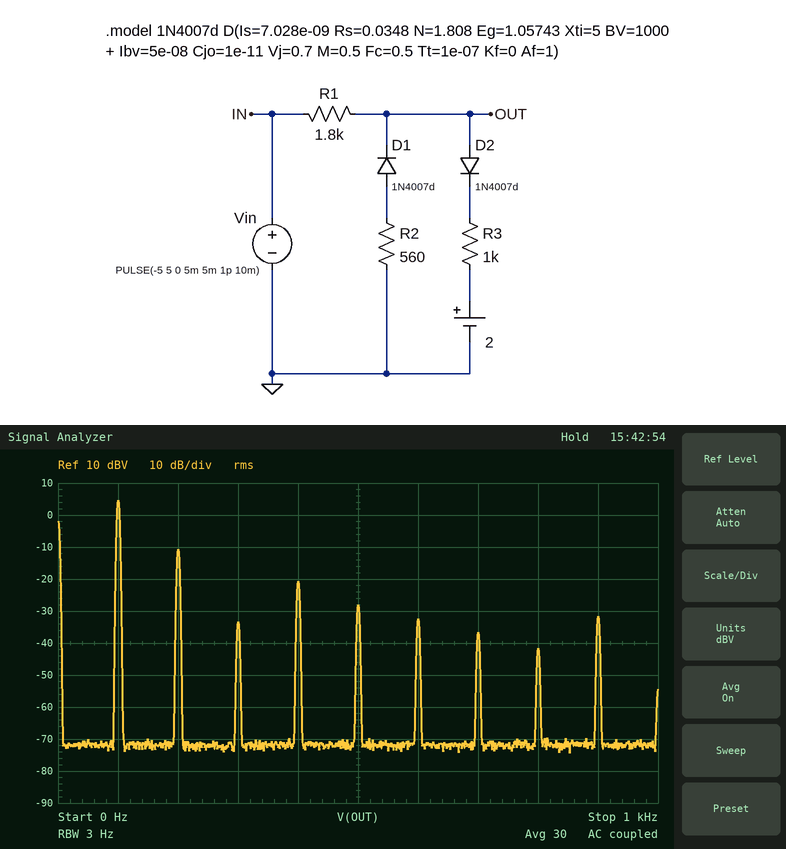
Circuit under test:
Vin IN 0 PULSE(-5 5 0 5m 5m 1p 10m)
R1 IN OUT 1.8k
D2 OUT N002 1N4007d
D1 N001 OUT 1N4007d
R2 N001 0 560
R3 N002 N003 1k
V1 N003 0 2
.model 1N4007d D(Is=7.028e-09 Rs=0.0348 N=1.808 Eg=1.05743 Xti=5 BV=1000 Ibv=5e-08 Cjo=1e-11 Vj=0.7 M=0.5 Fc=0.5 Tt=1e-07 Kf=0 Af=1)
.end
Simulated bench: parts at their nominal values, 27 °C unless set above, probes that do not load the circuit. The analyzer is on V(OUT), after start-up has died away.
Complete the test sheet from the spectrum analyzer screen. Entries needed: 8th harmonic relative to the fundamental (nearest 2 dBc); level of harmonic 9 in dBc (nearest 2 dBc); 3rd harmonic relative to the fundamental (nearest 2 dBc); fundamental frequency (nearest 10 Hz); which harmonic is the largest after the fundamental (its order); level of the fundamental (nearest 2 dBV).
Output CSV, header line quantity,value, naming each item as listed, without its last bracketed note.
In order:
quantity,value
8th harmonic relative to the fundamental,-46 dBc
level of harmonic 9 in dBc,-36 dBc
3rd harmonic relative to the fundamental,-38 dBc
fundamental frequency,100 Hz
which harmonic is the largest after the fundamental,2
level of the fundamental,4 dBV
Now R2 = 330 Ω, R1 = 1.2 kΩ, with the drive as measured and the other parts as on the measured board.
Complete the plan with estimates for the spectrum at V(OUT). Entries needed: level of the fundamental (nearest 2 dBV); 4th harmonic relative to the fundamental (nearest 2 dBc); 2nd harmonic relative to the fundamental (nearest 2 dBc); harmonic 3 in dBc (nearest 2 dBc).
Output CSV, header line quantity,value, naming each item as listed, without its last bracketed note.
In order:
quantity,value
level of the fundamental,4 dBV
4th harmonic relative to the fundamental,-28 dBc
2nd harmonic relative to the fundamental,-14 dBc
harmonic 3 in dBc,-58 dBc
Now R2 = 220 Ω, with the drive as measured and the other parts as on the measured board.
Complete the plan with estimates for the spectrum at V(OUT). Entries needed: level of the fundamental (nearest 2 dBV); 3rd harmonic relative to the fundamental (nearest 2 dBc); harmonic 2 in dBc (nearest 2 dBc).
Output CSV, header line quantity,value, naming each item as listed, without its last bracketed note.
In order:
quantity,value
level of the fundamental,4 dBV
3rd harmonic relative to the fundamental,-30 dBc
harmonic 2 in dBc,-12 dBc
